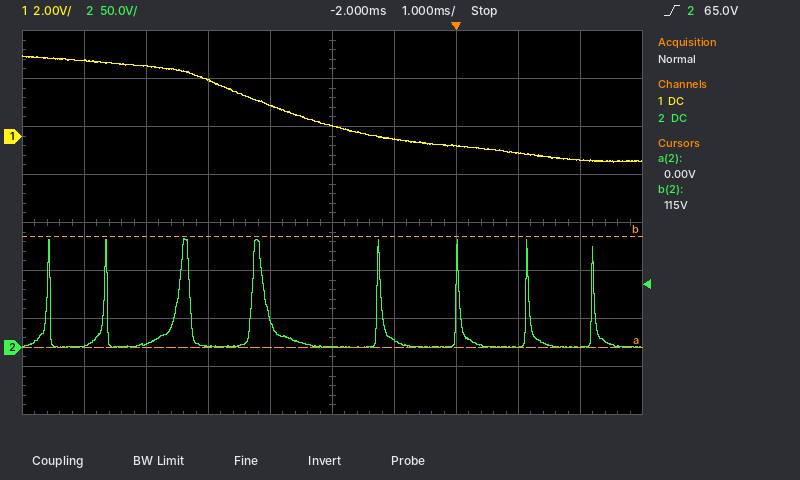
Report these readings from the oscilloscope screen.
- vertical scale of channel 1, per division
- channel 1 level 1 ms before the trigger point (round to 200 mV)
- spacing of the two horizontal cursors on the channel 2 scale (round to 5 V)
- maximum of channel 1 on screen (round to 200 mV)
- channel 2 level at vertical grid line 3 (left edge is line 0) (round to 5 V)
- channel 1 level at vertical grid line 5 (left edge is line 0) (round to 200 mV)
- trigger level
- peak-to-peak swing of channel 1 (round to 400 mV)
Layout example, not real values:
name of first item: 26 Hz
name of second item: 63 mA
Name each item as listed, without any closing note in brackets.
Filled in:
vertical scale of channel 1, per division: 2 V
channel 1 level 1 ms before the trigger point: -200 mV
spacing of the two horizontal cursors on the channel 2 scale: 115 V
maximum of channel 1 on screen: 3.4 V
channel 2 level at vertical grid line 3 (left edge is line 0): 0 V
channel 1 level at vertical grid line 5 (left edge is line 0): 400 mV
trigger level: 65.0 V
peak-to-peak swing of channel 1: 4.4 V
